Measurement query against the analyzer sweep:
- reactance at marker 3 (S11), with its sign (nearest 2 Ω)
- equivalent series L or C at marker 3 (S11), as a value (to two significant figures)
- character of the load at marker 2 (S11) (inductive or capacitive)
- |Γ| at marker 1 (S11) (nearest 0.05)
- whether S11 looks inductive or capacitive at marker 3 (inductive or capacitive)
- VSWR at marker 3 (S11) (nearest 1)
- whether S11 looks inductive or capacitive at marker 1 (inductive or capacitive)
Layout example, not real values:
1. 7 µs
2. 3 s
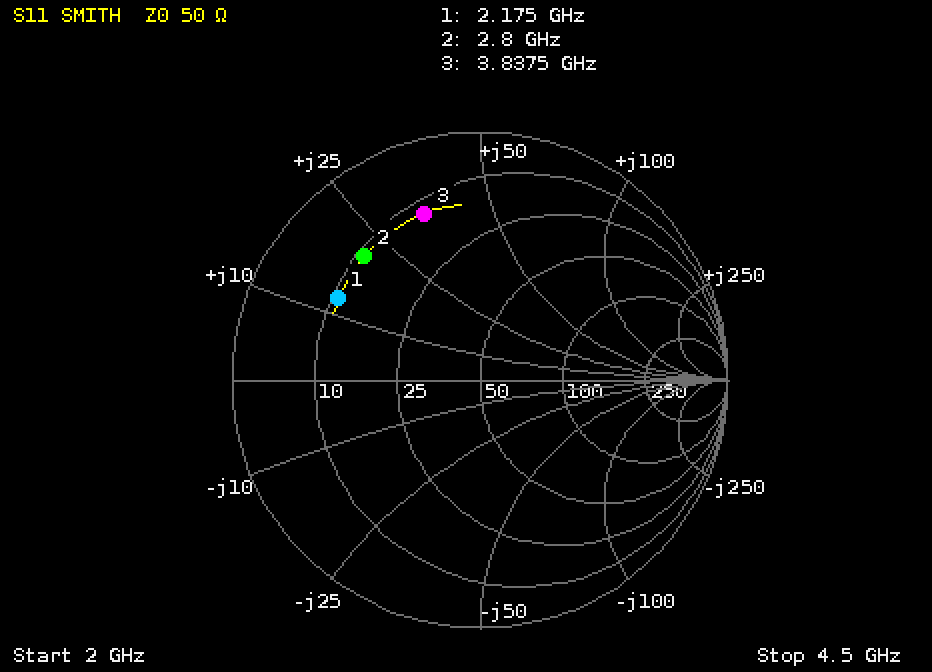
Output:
1. +34 Ω
2. 1.4 nH
3. inductive
4. 0.65
5. inductive
6. 6
7. inductive
